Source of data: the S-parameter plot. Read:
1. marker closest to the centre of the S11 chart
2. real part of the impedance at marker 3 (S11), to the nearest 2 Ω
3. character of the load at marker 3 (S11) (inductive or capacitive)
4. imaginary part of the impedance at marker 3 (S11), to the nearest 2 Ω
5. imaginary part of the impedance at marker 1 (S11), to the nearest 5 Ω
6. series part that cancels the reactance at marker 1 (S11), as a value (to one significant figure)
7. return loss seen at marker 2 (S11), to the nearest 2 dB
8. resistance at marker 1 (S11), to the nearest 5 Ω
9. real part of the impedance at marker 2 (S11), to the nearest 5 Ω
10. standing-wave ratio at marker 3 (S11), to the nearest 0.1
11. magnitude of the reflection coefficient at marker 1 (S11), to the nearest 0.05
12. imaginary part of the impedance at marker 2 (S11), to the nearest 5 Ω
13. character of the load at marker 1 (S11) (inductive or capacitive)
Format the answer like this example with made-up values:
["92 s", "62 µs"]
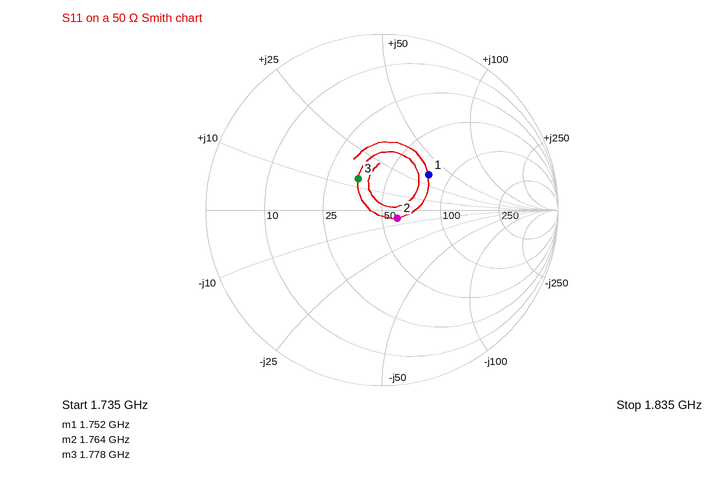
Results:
["marker 2", "36 Ω", "inductive", "+14 Ω", "+35 Ω", "3 pF", "20 dB", "75 Ω", "60 Ω", "1.6", "0.35", "-5 Ω", "inductive"]
